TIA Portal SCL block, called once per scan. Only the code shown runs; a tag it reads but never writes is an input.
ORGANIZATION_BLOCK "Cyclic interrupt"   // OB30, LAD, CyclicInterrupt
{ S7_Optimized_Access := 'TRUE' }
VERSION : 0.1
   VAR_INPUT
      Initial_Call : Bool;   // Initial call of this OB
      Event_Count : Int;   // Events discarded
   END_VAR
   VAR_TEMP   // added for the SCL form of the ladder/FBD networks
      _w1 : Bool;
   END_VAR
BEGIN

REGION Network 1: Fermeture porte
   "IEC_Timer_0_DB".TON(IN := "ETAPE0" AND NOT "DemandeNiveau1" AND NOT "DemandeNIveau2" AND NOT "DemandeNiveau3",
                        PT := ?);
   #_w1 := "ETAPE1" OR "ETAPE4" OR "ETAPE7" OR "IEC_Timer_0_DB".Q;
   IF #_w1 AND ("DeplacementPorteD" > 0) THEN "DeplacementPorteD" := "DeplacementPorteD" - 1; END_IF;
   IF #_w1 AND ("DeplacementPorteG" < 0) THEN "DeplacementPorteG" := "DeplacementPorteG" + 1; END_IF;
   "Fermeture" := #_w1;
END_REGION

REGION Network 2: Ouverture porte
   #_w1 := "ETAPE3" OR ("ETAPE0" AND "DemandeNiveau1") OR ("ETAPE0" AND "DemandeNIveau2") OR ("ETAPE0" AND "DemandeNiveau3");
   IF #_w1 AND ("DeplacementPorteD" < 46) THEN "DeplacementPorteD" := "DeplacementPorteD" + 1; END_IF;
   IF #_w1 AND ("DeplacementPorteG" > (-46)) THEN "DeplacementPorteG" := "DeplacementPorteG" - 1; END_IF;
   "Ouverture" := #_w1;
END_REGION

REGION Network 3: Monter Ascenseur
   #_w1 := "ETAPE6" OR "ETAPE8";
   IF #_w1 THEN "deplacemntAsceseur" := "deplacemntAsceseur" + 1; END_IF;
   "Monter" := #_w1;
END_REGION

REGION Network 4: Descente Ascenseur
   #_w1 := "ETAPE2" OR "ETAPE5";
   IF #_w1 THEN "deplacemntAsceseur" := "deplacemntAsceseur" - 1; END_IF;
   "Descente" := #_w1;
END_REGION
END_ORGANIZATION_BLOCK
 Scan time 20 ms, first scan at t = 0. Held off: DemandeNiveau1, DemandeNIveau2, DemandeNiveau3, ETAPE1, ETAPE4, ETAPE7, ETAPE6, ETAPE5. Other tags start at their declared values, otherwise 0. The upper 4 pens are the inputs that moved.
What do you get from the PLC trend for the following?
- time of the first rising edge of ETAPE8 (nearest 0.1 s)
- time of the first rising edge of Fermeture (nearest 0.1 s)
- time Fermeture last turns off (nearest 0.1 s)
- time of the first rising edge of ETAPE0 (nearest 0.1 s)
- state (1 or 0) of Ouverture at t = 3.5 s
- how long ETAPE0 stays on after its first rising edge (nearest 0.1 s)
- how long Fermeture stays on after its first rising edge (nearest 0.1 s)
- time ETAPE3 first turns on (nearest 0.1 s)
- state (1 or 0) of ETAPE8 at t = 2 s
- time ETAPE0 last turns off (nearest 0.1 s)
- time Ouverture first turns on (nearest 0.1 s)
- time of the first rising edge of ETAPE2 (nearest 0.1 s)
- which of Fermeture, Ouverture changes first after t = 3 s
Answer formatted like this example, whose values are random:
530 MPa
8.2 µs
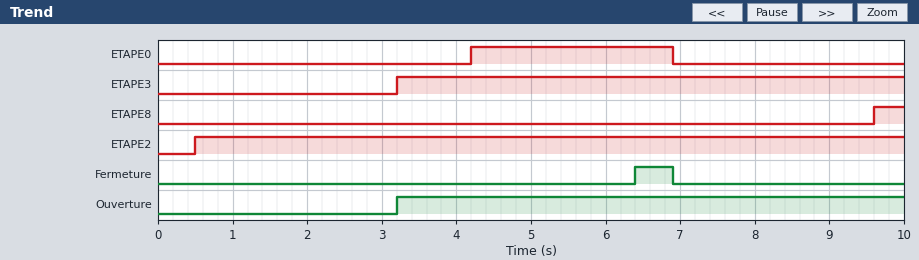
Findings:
9.6 s
6.4 s
6.9 s
4.2 s
1
2.7 s
0.5 s
3.2 s
0
6.9 s
3.2 s
0.5 s
Ouverture
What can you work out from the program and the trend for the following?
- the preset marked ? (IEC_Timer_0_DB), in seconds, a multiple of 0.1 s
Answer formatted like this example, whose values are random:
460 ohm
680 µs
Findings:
2.2 s
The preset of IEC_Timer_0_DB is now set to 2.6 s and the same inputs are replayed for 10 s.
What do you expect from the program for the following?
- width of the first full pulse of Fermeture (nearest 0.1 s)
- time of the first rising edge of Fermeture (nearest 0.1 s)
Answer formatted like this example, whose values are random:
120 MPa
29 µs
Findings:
0.1 s
6.8 s
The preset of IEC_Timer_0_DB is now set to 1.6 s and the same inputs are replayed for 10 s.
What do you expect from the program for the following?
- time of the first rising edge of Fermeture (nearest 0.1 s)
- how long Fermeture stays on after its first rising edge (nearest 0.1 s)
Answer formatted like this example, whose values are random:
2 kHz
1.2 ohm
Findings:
5.8 s
1.1 s
